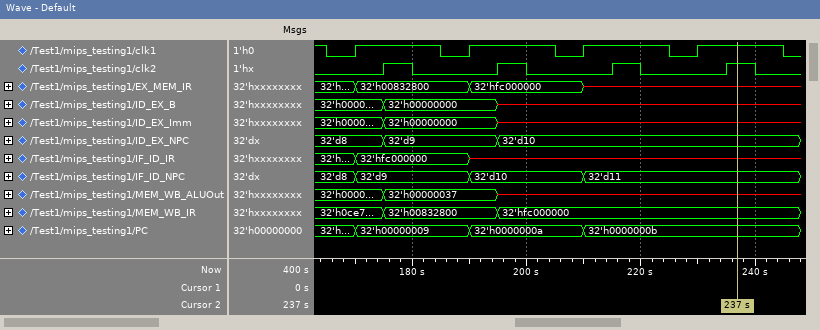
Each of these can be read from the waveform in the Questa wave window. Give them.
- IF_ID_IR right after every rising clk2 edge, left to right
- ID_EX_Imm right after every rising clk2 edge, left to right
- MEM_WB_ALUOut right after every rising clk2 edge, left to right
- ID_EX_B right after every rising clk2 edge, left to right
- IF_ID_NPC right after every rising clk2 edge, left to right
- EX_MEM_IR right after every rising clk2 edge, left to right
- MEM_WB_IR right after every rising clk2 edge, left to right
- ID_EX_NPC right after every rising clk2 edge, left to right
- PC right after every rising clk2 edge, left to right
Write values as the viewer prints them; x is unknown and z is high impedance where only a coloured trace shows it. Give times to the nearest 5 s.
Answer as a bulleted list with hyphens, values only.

- 32'hfc000000, x, x, x
- 32'h00000000, x, x, x
- 32'h00000037, x, x, x
- 32'h00000000, x, x, x
- 32'd9, 32'd10, 32'd11, 32'd11
- 32'h00832800, 32'hfc000000, x, x
- 32'h00832800, 32'hfc000000, 32'hfc000000, 32'hfc000000
- 32'd9, 32'd10, 32'd10, 32'd10
- 32'h00000009, 32'h0000000a, 32'h0000000b, 32'h0000000b
